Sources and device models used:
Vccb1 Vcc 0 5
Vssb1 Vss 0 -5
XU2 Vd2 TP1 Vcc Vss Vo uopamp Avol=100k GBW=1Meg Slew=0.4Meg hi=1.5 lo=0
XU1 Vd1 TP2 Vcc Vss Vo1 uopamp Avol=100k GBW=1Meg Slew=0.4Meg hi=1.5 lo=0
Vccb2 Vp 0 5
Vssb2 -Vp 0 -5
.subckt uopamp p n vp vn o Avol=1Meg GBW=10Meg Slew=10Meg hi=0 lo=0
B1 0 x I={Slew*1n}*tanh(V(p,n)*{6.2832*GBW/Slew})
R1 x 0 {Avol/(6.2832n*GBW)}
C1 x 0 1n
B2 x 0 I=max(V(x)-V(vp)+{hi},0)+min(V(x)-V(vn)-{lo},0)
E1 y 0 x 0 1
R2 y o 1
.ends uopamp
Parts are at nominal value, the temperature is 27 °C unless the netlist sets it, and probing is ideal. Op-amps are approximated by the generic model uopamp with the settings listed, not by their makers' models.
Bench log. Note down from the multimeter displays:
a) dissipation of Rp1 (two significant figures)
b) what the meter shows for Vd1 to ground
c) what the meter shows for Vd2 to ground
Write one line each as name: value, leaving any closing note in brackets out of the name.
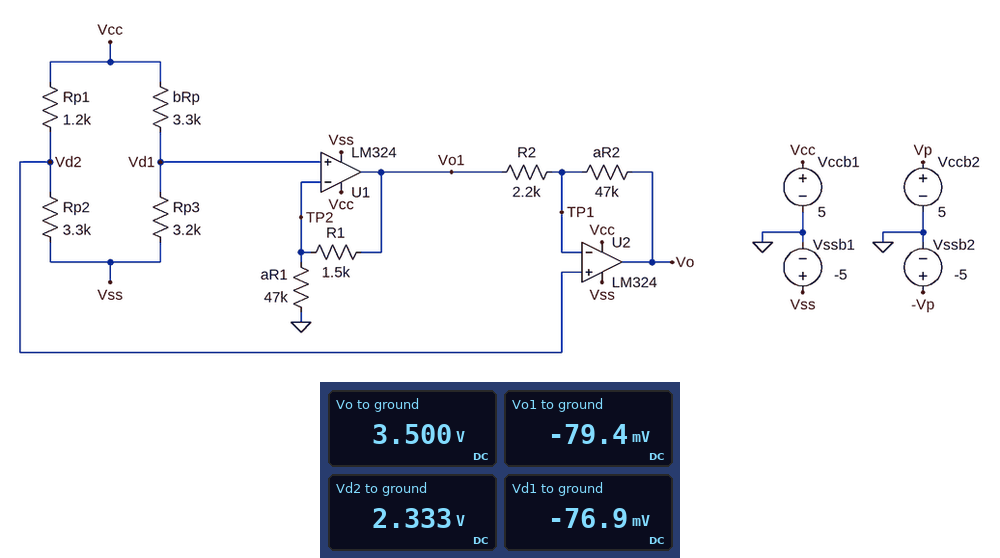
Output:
dissipation of Rp1: 5.9 mW
what the meter shows for Vd1 to ground: -76.9 mV
what the meter shows for Vd2 to ground: 2.333 V
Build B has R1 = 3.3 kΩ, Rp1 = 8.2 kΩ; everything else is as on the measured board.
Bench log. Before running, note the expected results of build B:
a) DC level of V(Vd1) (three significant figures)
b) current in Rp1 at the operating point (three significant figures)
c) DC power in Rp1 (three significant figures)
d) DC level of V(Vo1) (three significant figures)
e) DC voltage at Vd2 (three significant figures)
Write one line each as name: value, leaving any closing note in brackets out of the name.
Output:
DC level of V(Vd1): -76.9 mV
current in Rp1 at the operating point: 870 µA
DC power in Rp1: 6.20 mW
DC level of V(Vo1): -82.3 mV
DC voltage at Vd2: -2.13 V
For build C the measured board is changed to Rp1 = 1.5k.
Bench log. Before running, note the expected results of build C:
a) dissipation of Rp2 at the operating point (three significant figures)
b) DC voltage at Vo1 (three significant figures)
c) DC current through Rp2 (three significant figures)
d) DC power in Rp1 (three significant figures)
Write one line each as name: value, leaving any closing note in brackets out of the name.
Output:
dissipation of Rp2 at the operating point: 14.3 mW
DC voltage at Vo1: -79.4 mV
DC current through Rp2: 2.08 mA
DC power in Rp1: 6.51 mW
